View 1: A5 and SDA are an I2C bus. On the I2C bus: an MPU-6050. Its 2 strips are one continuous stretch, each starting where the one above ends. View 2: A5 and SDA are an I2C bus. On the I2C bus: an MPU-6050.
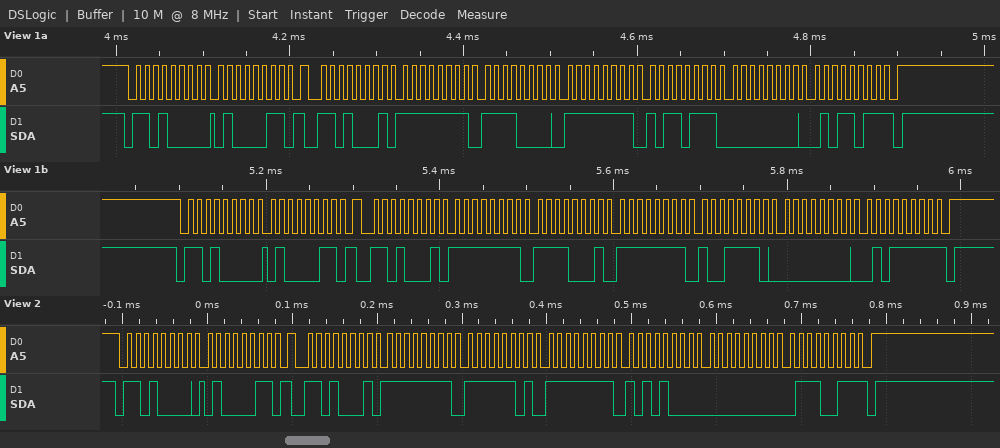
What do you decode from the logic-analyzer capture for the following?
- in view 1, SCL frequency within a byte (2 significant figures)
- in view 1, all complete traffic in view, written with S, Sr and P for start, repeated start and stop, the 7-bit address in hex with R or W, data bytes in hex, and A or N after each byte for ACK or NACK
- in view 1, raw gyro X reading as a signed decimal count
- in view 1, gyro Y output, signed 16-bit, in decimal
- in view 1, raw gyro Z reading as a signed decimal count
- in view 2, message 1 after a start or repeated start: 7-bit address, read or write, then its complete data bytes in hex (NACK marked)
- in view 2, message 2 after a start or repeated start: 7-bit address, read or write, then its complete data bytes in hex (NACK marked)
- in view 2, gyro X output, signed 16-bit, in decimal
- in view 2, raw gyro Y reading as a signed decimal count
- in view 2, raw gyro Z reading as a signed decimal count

100 kHz
S 68W A 43 A Sr 68R A FF A F0 A FF A B7 A 00 A 5B N P S 68W A 43 A Sr 68R A FF A F1 A FF A 9E A 00 A 5F N P
-16
-73
91
0x68 write: 43
0x68 read: FF FD FF A8 00 73 NACK
-3
-88
115
